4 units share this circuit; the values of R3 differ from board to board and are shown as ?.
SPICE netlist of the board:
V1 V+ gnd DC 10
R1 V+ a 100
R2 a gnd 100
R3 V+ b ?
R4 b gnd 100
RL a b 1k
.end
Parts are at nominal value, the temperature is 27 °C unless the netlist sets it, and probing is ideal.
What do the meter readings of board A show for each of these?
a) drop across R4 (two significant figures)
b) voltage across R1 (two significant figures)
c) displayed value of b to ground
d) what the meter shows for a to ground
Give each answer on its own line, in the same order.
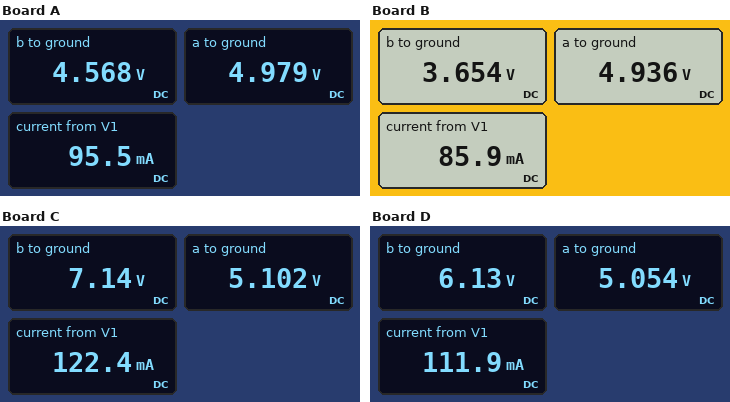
4.6 V
5.0 V
4.568 V
4.979 V
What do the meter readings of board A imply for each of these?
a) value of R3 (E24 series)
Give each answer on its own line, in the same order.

120 Ω
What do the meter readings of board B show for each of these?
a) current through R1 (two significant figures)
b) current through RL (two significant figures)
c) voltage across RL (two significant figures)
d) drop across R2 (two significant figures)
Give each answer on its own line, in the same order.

51 mA
1.3 mA
1.3 V
4.9 V
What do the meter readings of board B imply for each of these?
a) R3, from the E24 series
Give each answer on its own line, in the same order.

180 Ω
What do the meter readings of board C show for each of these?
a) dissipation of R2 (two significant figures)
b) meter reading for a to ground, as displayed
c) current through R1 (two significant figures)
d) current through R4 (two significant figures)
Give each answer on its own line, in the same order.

260 mW
5.102 V
49 mA
71 mA
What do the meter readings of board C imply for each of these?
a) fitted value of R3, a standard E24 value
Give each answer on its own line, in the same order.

39 Ω
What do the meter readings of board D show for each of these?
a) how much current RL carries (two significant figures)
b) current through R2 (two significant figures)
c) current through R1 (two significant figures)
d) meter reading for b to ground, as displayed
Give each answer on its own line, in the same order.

1.1 mA
51 mA
49 mA
6.13 V
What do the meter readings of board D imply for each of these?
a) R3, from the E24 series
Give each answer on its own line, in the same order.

62 Ω
